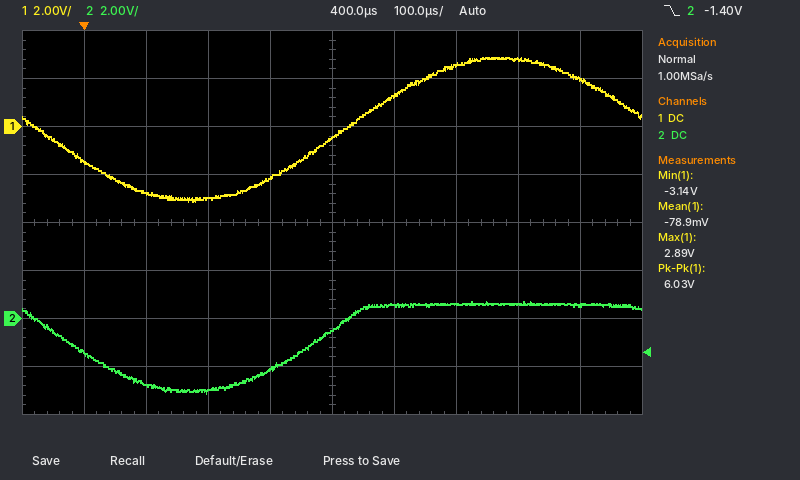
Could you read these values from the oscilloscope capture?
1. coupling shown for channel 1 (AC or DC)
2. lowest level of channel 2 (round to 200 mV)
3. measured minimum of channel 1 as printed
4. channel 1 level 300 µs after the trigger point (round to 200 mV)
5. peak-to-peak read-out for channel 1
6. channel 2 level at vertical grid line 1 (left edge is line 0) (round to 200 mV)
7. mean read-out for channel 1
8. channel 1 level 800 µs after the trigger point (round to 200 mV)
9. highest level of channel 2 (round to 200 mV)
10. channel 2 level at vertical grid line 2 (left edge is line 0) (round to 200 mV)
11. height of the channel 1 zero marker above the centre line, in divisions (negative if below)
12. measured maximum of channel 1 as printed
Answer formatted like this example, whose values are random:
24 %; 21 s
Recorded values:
DC; -3.2 V; -3.14 V; -2.2 V; 6.03 V; -1.4 V; -78.9 mV; 2.0 V; 800 mV; -2.8 V; +2.0 div; 2.89 V
